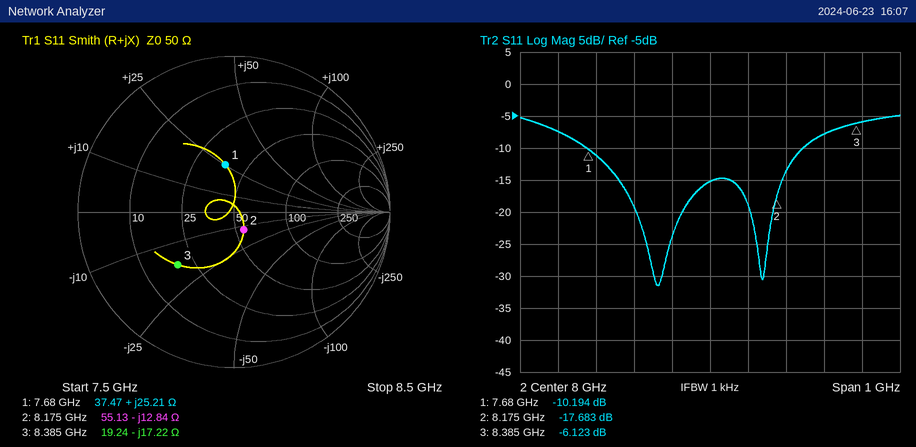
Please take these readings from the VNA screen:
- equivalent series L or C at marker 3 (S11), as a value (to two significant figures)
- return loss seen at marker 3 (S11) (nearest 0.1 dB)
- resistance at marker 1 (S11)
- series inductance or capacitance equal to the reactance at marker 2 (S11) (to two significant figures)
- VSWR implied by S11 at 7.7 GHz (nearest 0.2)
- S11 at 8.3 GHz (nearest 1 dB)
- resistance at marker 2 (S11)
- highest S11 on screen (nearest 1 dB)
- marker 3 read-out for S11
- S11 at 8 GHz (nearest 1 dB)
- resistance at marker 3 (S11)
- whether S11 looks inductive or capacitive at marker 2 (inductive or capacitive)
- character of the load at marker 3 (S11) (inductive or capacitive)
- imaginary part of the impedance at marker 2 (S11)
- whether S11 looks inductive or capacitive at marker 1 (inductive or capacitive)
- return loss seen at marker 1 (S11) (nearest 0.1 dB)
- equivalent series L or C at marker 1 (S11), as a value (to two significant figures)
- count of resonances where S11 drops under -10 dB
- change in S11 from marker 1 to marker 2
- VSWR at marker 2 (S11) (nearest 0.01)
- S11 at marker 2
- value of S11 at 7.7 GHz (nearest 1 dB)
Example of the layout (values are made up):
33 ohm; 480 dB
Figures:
1.1 pF; 6.1 dB; 37.47 Ω; 1.5 pF; 1.8; -8 dB; 55.13 Ω; -5 dB; -6.123 dB; -15 dB; 19.24 Ω; capacitive; capacitive; -12.84 Ω; inductive; 10.2 dB; 520 pH; 2; -7.489 dB; 1.30; -17.683 dB; -11 dB
